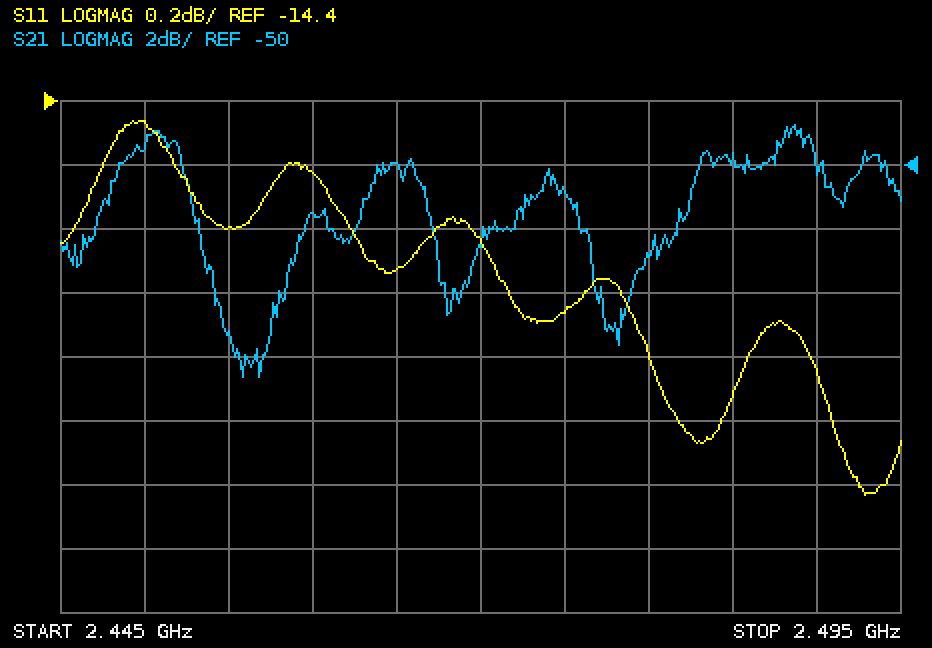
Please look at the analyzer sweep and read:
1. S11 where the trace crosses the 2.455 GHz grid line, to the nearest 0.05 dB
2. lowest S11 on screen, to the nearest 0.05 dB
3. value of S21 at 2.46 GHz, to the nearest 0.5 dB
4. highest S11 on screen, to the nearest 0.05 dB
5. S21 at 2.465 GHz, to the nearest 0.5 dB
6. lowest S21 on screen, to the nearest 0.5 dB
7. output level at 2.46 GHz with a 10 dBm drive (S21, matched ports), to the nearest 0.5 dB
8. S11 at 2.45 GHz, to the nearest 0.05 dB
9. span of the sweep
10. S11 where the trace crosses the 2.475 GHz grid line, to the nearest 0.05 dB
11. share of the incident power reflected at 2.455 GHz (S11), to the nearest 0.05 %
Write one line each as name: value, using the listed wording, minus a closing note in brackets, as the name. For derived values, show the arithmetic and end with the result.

S11 where the trace crosses the 2.455 GHz grid line, to the nearest 0.05 dB: -14.80 dB
lowest S11 on screen, to the nearest 0.05 dB: -15.65 dB
value of S21 at 2.46 GHz, to the nearest 0.5 dB: -51.5 dB
highest S11 on screen, to the nearest 0.05 dB: -14.45 dB
S21 at 2.465 GHz, to the nearest 0.5 dB: -50.0 dB
lowest S21 on screen, to the nearest 0.5 dB: -56.5 dB
output level at 2.46 GHz with a 10 dBm drive (S21, matched ports), to the nearest 0.5 dB: 10 dBm + (-51.5 dB) = -41.5 dBm
S11 at 2.45 GHz, to the nearest 0.05 dB: -14.45 dB
span of the sweep: 50 MHz
S11 where the trace crosses the 2.475 GHz grid line, to the nearest 0.05 dB: -15.05 dB
share of the incident power reflected at 2.455 GHz (S11), to the nearest 0.05 %: 10^(-14.8/10) ≈ 3.31 %, so 3.30 % to the nearest 0.05 %
